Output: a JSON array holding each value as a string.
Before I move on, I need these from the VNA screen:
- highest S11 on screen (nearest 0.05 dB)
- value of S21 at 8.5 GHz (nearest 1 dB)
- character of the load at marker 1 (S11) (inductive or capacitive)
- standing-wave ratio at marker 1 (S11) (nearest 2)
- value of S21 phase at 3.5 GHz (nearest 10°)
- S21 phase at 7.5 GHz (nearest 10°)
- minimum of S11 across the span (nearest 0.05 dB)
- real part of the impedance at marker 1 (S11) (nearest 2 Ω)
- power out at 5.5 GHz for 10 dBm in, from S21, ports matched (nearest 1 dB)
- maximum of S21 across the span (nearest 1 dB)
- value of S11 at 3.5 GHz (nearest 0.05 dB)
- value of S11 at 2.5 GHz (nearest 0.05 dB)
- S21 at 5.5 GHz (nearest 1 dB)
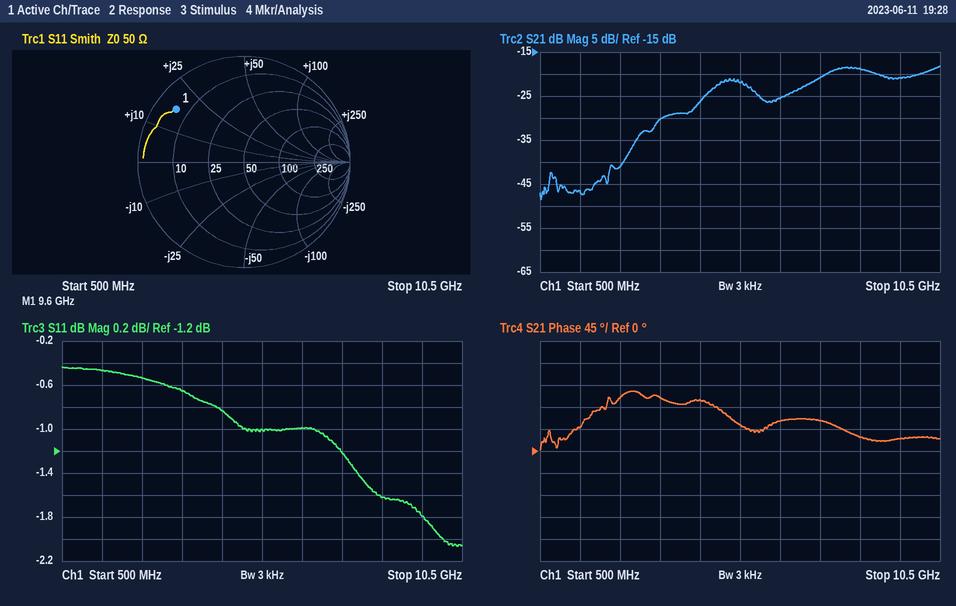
["-0.45 dB", "-19 dB", "inductive", "10", "110°", "60°", "-2.05 dB", "6 Ω", "-12 dBm", "-18 dB", "-0.65 dB", "-0.55 dB", "-22 dB"]
